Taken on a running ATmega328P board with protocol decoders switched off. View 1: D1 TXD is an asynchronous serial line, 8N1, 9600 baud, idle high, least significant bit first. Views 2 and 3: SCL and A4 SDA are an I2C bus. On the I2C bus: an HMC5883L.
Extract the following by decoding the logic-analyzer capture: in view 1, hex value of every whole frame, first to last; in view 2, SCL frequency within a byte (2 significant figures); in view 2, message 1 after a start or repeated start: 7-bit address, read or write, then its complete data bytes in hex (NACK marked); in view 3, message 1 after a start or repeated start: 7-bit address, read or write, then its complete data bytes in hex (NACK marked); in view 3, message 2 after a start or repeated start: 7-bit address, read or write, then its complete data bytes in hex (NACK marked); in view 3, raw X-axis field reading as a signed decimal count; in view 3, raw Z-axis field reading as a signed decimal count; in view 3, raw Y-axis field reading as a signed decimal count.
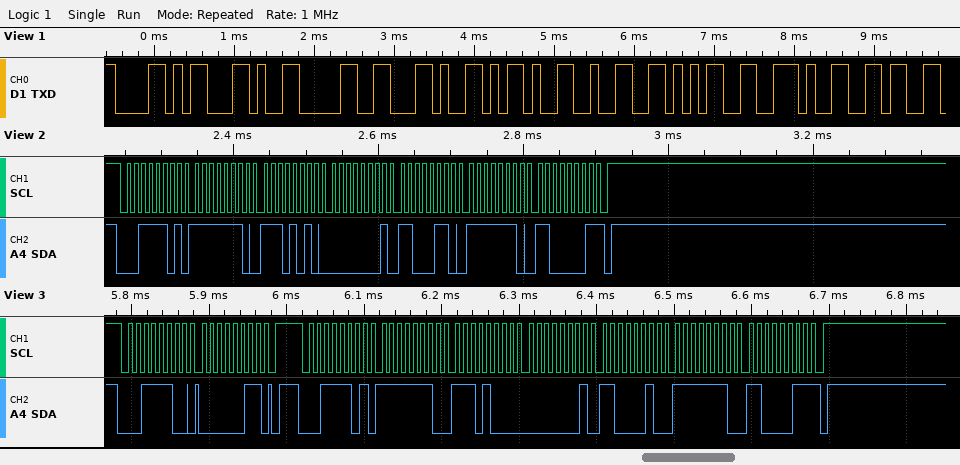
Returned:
58 2C 30 2C 2D 32 35 2E 36
100 kHz
0x1E read: FE EA 01 C6 FE C1 NACK
0x1E write: 03
0x1E read: FE E8 01 C2 FE C3 NACK
-280
450
-317
